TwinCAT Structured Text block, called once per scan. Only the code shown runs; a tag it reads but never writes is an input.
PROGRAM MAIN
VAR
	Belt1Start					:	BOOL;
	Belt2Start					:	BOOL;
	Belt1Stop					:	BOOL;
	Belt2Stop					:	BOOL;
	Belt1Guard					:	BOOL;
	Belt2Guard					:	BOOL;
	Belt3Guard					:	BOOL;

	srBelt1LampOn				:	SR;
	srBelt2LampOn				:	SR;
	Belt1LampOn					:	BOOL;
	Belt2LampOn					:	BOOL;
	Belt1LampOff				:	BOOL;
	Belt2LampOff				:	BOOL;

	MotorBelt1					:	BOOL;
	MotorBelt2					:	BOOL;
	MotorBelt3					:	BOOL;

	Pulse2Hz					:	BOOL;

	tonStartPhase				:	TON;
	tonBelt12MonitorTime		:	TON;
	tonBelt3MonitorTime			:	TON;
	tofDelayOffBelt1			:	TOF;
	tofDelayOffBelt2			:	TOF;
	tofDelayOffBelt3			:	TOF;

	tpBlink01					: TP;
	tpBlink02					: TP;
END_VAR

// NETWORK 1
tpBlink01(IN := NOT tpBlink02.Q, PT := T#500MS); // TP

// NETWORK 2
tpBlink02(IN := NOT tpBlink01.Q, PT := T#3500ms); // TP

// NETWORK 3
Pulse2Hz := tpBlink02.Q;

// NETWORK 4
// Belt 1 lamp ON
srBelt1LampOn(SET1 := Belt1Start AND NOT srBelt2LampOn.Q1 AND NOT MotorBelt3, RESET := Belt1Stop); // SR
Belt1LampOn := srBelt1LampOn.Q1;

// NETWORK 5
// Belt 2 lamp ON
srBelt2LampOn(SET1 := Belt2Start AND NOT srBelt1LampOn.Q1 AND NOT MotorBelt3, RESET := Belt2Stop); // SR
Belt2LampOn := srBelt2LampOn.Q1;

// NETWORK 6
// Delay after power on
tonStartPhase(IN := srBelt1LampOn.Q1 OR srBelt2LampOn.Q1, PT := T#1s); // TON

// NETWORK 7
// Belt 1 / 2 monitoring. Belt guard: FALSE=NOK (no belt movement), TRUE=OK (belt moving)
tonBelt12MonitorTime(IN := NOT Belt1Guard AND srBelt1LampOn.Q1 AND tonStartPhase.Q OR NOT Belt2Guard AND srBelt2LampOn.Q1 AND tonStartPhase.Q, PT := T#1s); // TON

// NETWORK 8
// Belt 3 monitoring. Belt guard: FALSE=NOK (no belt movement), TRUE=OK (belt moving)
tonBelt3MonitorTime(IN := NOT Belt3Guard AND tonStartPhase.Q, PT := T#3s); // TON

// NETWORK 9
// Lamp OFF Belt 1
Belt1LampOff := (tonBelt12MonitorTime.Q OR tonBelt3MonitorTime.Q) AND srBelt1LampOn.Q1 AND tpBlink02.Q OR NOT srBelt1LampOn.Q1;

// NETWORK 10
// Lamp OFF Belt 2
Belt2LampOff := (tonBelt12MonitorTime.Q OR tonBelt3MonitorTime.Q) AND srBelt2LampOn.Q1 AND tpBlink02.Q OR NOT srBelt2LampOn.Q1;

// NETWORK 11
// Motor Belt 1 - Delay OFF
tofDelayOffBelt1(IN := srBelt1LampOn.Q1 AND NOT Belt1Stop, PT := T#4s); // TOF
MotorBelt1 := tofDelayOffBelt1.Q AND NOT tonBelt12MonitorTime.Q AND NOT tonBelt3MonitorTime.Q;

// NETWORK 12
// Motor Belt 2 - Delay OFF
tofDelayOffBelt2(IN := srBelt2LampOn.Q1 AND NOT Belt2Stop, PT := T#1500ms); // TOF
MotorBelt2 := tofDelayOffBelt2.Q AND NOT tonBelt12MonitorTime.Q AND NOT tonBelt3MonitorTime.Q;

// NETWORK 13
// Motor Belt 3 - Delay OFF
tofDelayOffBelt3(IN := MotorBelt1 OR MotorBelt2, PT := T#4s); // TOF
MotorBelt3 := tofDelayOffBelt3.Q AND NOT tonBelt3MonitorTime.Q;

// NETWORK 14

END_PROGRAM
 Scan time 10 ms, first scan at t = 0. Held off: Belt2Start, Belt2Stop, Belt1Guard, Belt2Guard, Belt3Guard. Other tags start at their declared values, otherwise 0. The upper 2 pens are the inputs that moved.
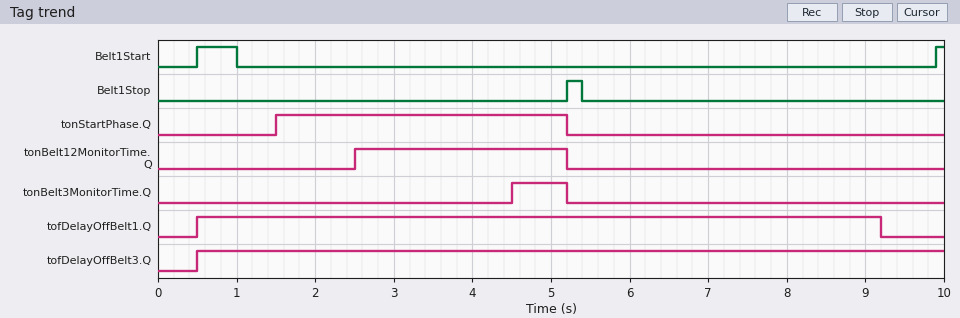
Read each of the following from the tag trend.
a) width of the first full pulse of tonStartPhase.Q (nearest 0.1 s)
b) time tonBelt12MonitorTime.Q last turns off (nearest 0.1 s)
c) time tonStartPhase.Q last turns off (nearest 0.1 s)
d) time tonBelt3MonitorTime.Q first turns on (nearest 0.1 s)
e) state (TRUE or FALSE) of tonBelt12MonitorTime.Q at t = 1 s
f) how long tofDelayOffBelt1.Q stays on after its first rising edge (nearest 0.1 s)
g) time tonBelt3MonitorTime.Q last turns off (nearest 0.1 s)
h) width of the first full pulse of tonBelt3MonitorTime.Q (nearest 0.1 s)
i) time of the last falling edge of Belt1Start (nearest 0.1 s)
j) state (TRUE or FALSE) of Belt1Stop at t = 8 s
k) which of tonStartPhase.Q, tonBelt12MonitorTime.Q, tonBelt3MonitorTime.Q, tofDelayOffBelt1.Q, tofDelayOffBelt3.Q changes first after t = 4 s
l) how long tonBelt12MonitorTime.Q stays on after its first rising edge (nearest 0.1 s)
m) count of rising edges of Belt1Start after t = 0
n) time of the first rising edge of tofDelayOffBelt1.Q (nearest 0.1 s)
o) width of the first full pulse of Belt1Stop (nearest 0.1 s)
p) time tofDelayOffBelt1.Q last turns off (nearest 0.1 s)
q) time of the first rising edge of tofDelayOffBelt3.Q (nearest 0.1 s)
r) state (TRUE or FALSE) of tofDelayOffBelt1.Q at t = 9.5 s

3.7 s
5.2 s
5.2 s
4.5 s
FALSE
8.7 s
5.2 s
0.7 s
1.0 s
FALSE
tonBelt3MonitorTime.Q
2.7 s
2
0.5 s
0.2 s
9.2 s
0.5 s
FALSE
